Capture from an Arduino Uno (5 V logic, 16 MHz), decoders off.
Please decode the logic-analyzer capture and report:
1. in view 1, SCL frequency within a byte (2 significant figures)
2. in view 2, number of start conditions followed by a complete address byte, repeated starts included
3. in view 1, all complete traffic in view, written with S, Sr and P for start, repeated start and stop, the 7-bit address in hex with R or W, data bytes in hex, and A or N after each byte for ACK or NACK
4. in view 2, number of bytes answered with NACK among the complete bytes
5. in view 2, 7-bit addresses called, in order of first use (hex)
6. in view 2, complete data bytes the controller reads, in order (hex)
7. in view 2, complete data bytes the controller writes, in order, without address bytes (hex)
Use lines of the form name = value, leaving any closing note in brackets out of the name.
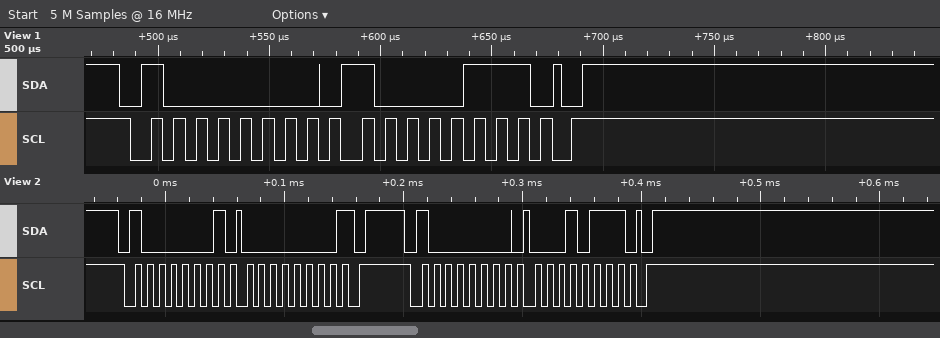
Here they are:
in view 1, SCL frequency within a byte = 100 kHz
in view 2, number of start conditions followed by a complete address byte, repeated starts included = 2
in view 1, all complete traffic in view, written with S, Sr and P for start, repeated start and stop, the 7-bit address in hex with R or W, data bytes in hex, and A or N after each byte for ACK or NACK = S 40W A 87 A P
in view 2, number of bytes answered with NACK among the complete bytes = 1
in view 2, 7-bit addresses called, in order of first use = 0x40
in view 2, complete data bytes the controller reads, in order = 00
in view 2, complete data bytes the controller writes, in order, without address bytes = 17
